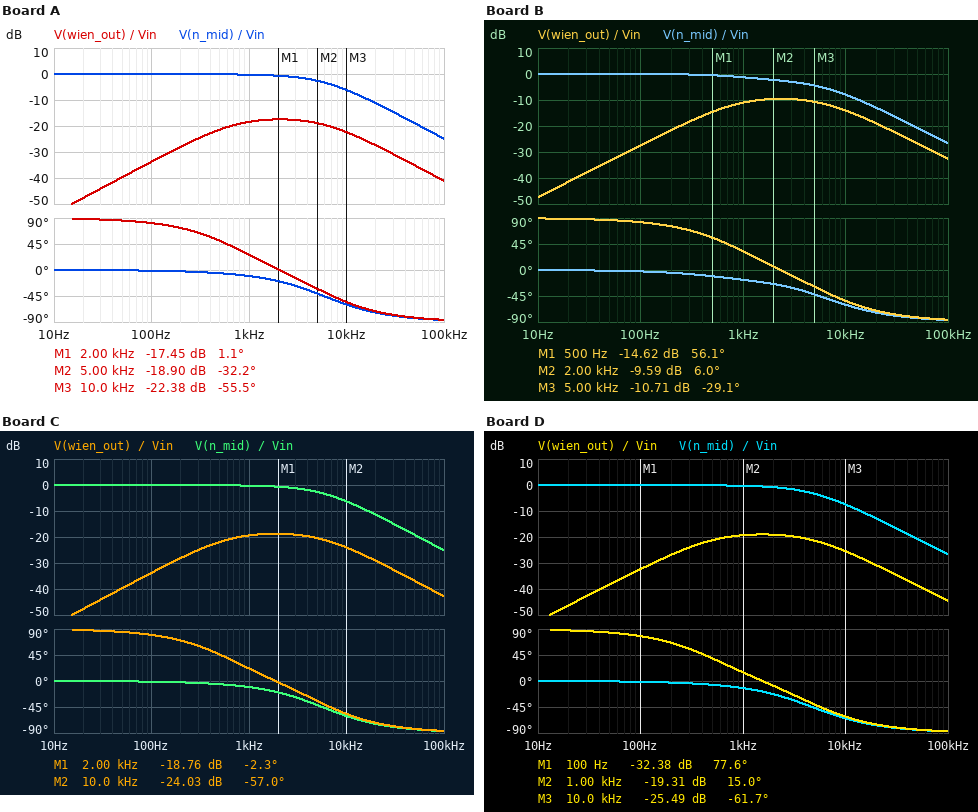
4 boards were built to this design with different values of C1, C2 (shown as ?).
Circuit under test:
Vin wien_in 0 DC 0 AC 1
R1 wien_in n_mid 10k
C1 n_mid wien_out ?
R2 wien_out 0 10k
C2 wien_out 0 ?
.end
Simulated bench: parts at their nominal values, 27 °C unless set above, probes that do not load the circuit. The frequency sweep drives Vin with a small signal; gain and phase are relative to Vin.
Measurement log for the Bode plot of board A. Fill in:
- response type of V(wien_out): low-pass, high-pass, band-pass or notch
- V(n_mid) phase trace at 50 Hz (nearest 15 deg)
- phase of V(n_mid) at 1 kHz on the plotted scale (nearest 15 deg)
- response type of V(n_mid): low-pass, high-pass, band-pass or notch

band-pass
0 deg
-15 deg
low-pass
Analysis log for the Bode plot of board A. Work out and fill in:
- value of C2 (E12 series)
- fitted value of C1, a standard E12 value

18 nF
3.3 nF
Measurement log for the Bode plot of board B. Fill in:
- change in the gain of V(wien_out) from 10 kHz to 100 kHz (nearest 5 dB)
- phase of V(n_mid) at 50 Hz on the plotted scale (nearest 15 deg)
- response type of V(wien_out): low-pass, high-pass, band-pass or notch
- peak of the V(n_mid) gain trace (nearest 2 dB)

-20 dB
0 deg
band-pass
0 dB
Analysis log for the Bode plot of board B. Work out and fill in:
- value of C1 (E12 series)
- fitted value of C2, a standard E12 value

6.8 nF
6.8 nF
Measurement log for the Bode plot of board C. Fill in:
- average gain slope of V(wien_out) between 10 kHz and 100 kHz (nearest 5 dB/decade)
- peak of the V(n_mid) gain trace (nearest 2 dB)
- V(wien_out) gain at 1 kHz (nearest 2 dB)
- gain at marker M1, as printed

-20 dB/decade
0 dB
-20 dB
-18.76 dB
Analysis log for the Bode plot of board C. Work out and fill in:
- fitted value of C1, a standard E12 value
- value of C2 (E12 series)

3.3 nF
22 nF
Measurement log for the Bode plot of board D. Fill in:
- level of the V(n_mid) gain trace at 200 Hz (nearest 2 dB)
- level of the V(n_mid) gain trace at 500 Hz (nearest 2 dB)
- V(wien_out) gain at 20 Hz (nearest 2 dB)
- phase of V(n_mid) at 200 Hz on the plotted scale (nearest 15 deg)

0 dB
0 dB
-46 dB
0 deg
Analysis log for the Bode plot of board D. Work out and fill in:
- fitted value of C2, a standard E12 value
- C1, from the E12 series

27 nF
3.9 nF
